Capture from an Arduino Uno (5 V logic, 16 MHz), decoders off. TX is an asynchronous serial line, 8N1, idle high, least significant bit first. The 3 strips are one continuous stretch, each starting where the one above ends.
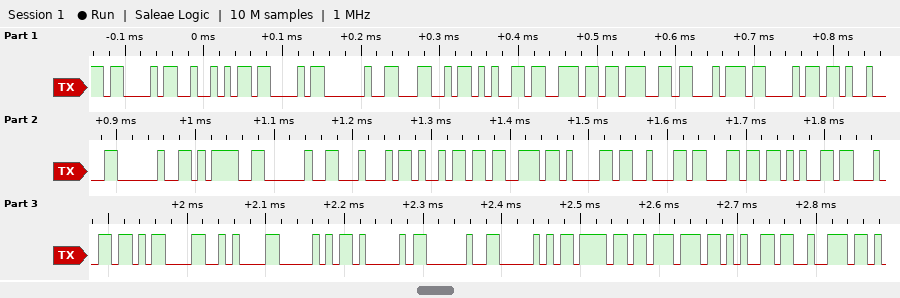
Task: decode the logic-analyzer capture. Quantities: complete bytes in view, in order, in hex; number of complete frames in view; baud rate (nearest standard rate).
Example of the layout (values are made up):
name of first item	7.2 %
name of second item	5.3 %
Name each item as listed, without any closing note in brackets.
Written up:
complete bytes in view, in order, in hex	43 52 43 20 4C 65 6E 67 74 68 09 20 3D 20 44 69 73 61 62 6C 65 64 0D 0A 50 41 20 50 6F 77 65 72
number of complete frames in view	32
baud rate	115200 baud
